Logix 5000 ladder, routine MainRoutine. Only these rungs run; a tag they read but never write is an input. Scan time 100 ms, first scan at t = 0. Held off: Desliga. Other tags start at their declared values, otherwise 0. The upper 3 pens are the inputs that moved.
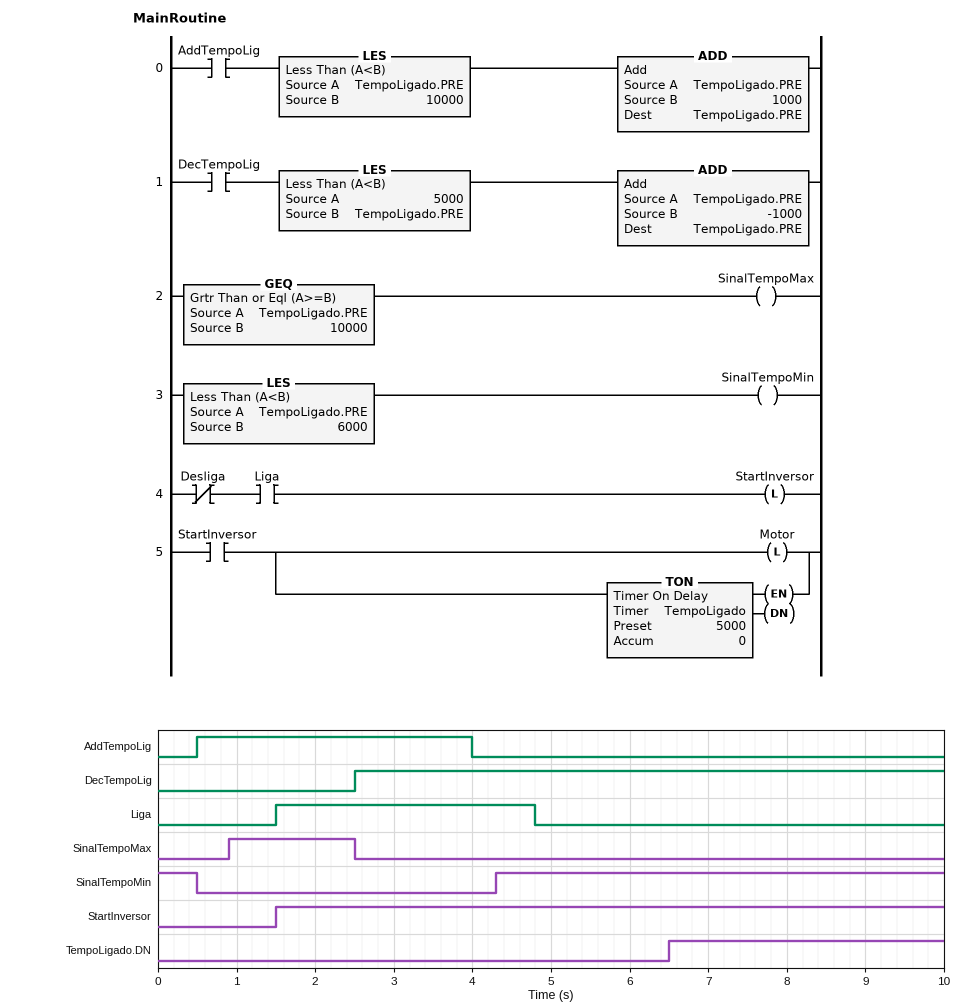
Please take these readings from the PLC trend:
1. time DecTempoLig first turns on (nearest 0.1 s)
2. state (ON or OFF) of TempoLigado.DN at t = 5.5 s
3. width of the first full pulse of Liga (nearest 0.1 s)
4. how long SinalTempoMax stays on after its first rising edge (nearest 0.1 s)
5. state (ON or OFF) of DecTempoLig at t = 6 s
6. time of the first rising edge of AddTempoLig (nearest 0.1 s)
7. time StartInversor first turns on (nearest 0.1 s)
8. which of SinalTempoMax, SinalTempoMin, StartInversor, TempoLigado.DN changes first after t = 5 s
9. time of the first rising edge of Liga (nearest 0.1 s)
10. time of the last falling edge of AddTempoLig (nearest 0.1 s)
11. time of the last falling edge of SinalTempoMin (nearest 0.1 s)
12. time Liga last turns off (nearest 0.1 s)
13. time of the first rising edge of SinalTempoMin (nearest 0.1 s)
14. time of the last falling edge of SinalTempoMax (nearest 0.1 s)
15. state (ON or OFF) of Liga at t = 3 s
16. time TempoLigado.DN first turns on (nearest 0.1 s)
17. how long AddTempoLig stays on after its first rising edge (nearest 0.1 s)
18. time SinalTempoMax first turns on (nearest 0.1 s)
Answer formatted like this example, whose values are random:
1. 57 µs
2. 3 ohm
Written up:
1. 2.5 s
2. OFF
3. 3.3 s
4. 1.6 s
5. ON
6. 0.5 s
7. 1.5 s
8. TempoLigado.DN
9. 1.5 s
10. 4.0 s
11. 0.5 s
12. 4.8 s
13. 4.3 s
14. 2.5 s
15. ON
16. 6.5 s
17. 3.5 s
18. 0.9 s
